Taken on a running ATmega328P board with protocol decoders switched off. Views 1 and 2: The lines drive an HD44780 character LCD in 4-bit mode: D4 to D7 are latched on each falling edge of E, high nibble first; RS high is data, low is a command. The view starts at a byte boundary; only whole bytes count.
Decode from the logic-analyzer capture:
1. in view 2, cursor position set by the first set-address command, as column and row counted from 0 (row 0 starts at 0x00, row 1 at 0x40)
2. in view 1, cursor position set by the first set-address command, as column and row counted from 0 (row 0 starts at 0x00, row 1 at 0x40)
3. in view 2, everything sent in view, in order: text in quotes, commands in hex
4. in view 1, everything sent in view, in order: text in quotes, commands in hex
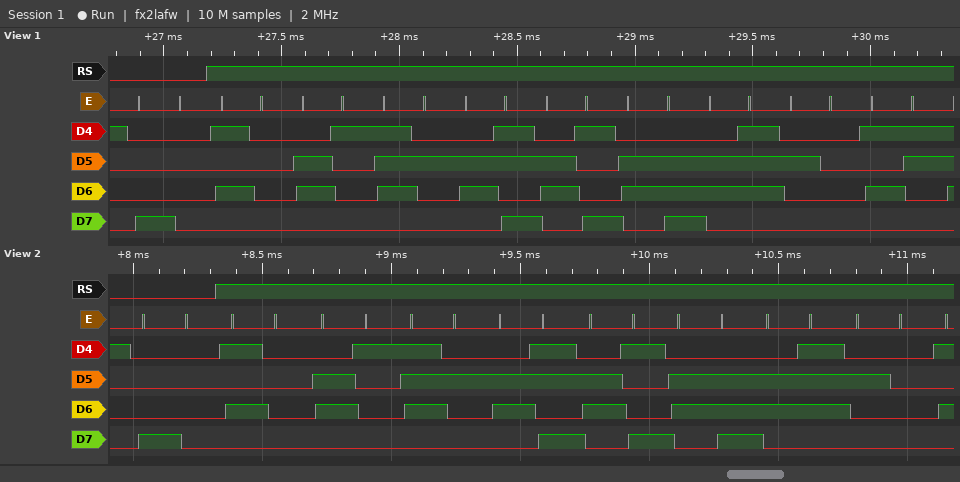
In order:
column 0, row 0
column 0, row 0
0x80 "Parking "
0x80 "Parking S"
